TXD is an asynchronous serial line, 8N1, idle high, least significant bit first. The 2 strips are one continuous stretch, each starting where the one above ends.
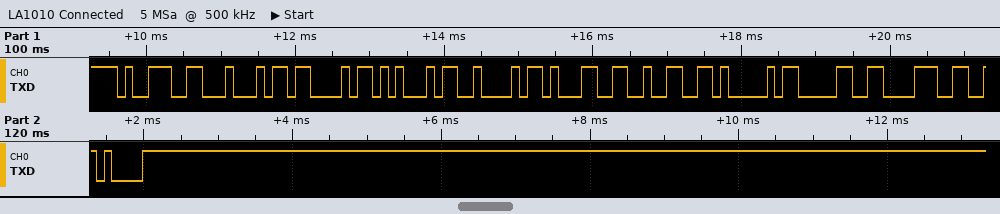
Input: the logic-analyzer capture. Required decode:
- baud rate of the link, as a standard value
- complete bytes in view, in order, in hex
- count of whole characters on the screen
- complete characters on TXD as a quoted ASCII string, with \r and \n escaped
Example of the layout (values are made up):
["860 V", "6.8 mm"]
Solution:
["9600 baud", "0x39 0x44 0x43 0x45 0x42 0x31 0x32 0x41 0x30 0x38 0x0A", "11", "\"9DCEB12A08\\n\""]
